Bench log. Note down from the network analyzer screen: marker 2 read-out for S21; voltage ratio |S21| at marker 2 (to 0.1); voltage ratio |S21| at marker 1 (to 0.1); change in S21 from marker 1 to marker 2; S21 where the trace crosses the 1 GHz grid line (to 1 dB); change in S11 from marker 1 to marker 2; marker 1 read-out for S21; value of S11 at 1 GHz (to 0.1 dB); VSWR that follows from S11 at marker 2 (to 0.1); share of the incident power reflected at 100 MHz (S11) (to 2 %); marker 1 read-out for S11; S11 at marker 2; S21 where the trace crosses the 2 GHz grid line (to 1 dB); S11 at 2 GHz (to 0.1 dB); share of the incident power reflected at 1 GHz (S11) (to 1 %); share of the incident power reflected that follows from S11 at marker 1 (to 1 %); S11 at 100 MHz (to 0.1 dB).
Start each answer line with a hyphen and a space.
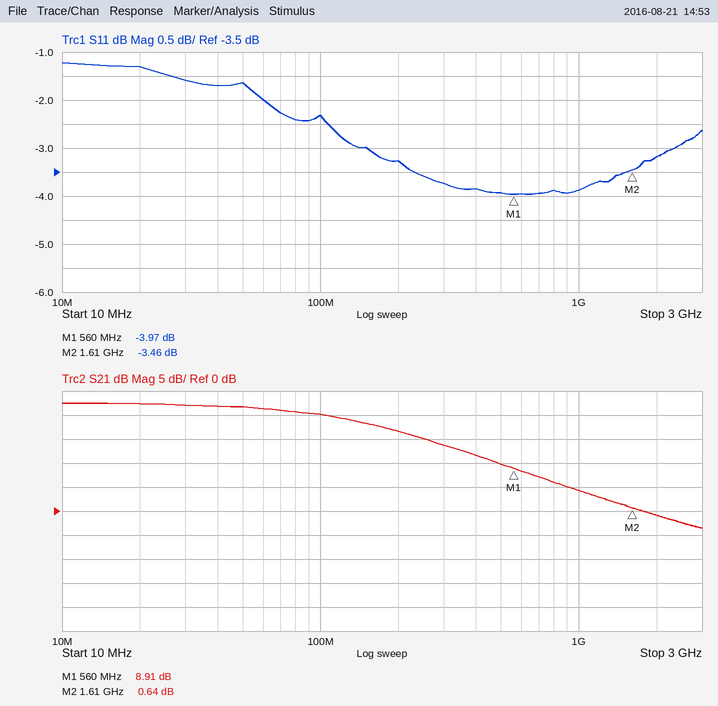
- 0.64 dB
- 1.1
- 2.8
- -8.27 dB
- 4 dB
- 0.51 dB
- 8.91 dB
- -3.9 dB
- 5.1
- 58 %
- -3.97 dB
- -3.46 dB
- -1 dB
- -3.2 dB
- 41 %
- 40 %
- -2.3 dB
